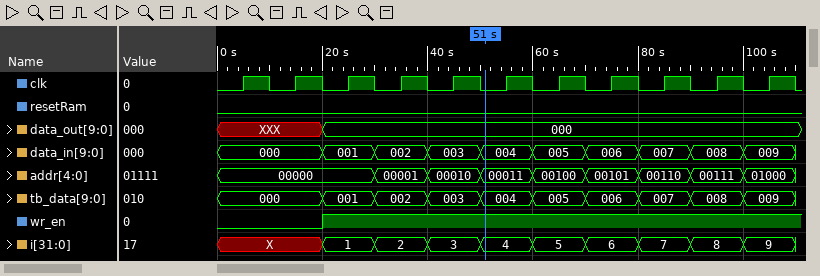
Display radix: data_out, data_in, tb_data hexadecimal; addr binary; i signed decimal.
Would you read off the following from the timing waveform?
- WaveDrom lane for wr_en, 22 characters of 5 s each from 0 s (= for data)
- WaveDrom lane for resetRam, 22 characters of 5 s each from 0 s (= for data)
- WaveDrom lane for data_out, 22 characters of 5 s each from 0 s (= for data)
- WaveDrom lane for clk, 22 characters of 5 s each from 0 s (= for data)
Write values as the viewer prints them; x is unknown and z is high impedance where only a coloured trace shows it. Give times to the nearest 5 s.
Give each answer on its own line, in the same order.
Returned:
{name: 'wr_en', wave: '0...1.................'}
{name: 'resetRam', wave: '0.....................'}
{name: 'data_out', wave: 'x...=.................', data: '000'}
{name: 'clk', wave: '0101010101010101010101'}
